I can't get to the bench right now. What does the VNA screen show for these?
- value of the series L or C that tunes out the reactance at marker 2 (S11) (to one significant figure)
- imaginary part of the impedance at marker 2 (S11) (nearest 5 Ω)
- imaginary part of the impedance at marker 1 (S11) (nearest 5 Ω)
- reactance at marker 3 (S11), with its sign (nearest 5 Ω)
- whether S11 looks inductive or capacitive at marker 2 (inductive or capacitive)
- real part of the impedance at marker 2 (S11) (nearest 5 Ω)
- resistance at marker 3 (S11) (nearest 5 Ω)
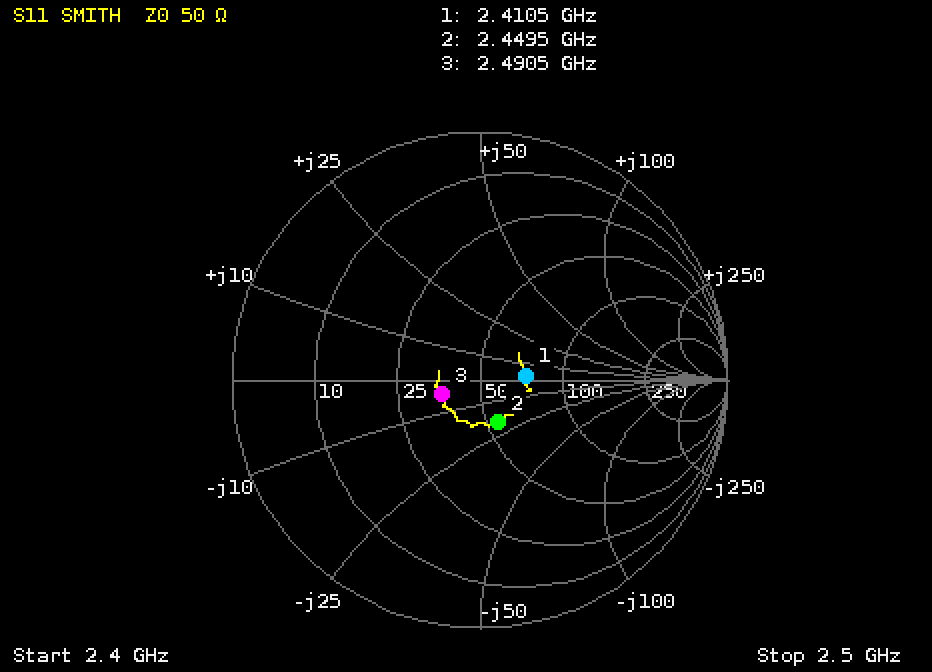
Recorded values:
1 nH
-20 Ω
+5 Ω
-5 Ω
capacitive
55 Ω
35 Ω
